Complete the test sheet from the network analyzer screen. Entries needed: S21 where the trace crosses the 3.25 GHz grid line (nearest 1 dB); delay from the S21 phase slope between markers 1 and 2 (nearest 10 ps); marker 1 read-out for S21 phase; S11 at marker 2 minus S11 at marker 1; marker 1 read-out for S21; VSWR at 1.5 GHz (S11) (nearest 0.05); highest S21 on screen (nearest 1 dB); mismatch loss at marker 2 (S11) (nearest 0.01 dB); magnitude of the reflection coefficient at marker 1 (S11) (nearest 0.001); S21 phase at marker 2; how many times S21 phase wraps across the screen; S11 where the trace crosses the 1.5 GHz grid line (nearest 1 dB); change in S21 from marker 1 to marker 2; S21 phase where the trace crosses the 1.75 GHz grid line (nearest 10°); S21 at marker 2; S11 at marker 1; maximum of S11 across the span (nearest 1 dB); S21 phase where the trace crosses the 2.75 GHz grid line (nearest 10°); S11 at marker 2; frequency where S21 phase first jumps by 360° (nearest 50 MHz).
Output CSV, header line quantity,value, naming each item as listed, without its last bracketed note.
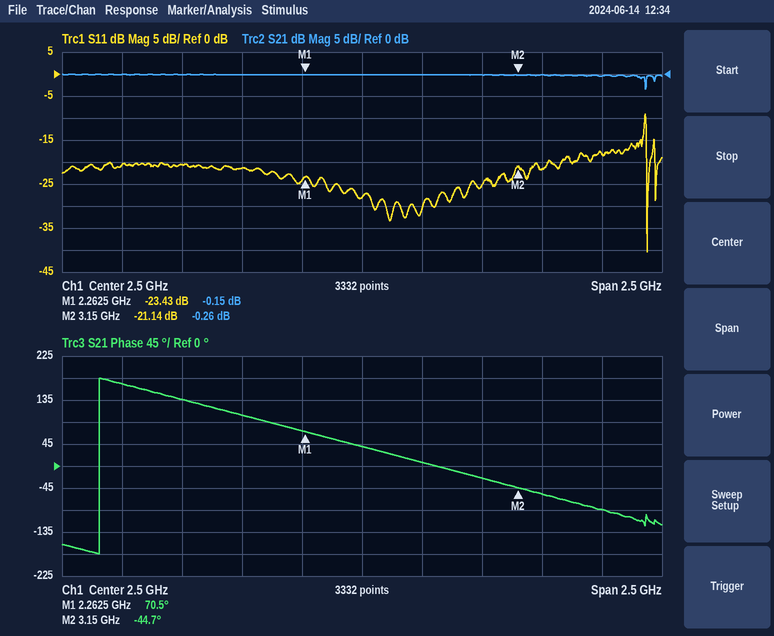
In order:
quantity,value
S21 where the trace crosses the 3.25 GHz grid line,0 dB
delay from the S21 phase slope between markers 1 and 2,360 ps
marker 1 read-out for S21 phase,70.5°
S11 at marker 2 minus S11 at marker 1,2.29 dB
marker 1 read-out for S21,-0.15 dB
VSWR at 1.5 GHz (S11),1.20
highest S21 on screen,0 dB
mismatch loss at marker 2 (S11),0.03 dB
magnitude of the reflection coefficient at marker 1 (S11),0.067
S21 phase at marker 2,-44.7°
how many times S21 phase wraps across the screen,1
S11 where the trace crosses the 1.5 GHz grid line,-21 dB
change in S21 from marker 1 to marker 2,-0.11 dB
S21 phase where the trace crosses the 1.75 GHz grid line,140°
S21 at marker 2,-0.26 dB
S11 at marker 1,-23.43 dB
maximum of S11 across the span,-9 dB
S21 phase where the trace crosses the 2.75 GHz grid line,10°
S11 at marker 2,-21.14 dB
frequency where S21 phase first jumps by 360°,1.40 GHz
